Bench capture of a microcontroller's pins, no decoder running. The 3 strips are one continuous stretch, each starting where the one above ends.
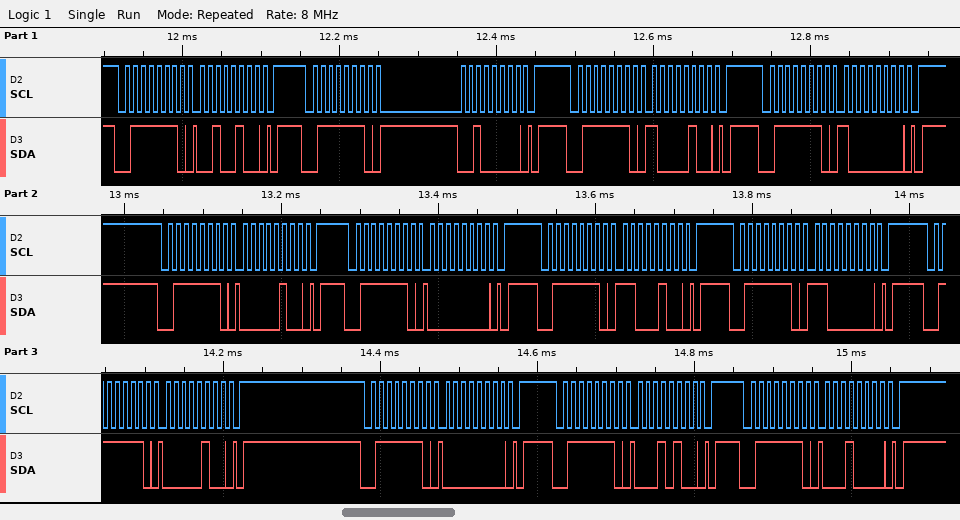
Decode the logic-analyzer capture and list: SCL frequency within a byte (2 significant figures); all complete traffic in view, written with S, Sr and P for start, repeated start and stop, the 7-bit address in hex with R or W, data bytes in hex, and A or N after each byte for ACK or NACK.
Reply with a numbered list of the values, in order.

1. 100 kHz
2. S 3FW A 24 A P S 3FW A 20 A P S 3FW A 84 A P S 3FW A 80 A P S 3FW A 04 A P S 3FW A 00 A P S 3FW A C4 A P S 3FW A C0 A P S 3FW A 04 A P S 3FW A 00 A P S 3FW A 14 A P S 3FW A 10 A P
